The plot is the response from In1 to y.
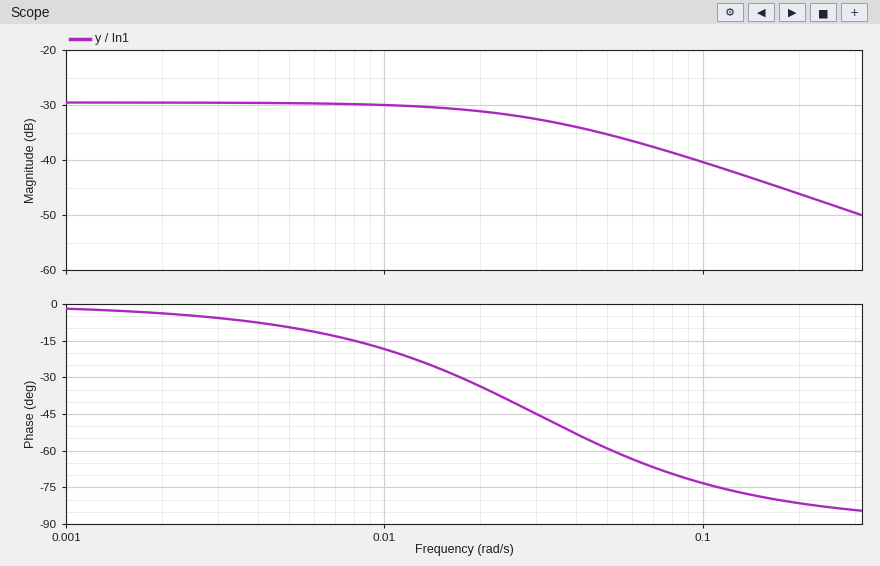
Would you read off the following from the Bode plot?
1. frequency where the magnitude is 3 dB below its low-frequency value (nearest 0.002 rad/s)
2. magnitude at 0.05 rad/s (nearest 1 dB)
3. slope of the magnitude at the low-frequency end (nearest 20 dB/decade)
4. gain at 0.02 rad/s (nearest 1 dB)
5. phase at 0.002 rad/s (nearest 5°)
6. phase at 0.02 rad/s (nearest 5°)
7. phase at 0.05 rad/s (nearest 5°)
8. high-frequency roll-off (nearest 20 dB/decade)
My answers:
0.030 rad/s
-35 dB
0 dB/decade
-31 dB
-5°
-35°
-60°
-20 dB/decade
